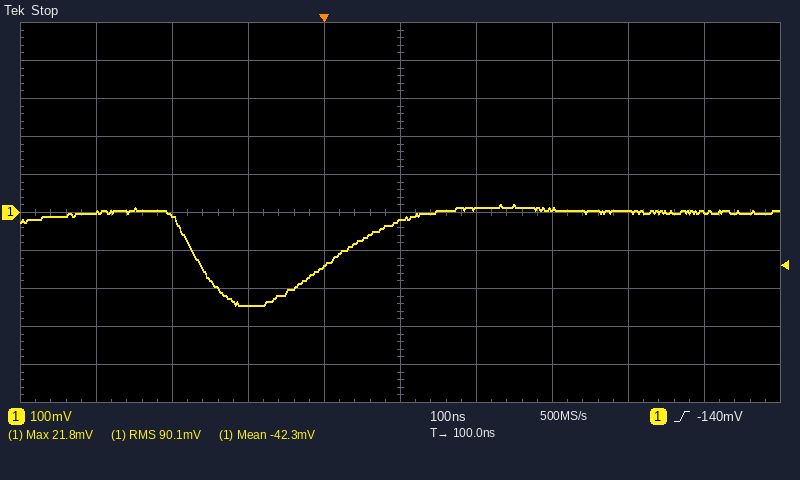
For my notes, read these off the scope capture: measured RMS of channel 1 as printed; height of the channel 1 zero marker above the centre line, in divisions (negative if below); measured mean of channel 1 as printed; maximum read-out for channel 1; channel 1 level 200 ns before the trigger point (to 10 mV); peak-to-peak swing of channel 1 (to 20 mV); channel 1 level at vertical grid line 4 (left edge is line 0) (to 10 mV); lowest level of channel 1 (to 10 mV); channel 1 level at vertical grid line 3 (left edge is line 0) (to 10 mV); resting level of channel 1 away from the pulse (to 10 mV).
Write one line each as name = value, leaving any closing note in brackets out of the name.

measured RMS of channel 1 as printed = 90.1 mV
height of the channel 1 zero marker above the centre line, in divisions = 0.0 div
measured mean of channel 1 as printed = -42.3 mV
maximum read-out for channel 1 = 21.8 mV
channel 1 level 200 ns before the trigger point = -10 mV
peak-to-peak swing of channel 1 = 260 mV
channel 1 level at vertical grid line 4 (left edge is line 0) = -140 mV
lowest level of channel 1 = -240 mV
channel 1 level at vertical grid line 3 (left edge is line 0) = -240 mV
resting level of channel 1 away from the pulse = 0 mV
